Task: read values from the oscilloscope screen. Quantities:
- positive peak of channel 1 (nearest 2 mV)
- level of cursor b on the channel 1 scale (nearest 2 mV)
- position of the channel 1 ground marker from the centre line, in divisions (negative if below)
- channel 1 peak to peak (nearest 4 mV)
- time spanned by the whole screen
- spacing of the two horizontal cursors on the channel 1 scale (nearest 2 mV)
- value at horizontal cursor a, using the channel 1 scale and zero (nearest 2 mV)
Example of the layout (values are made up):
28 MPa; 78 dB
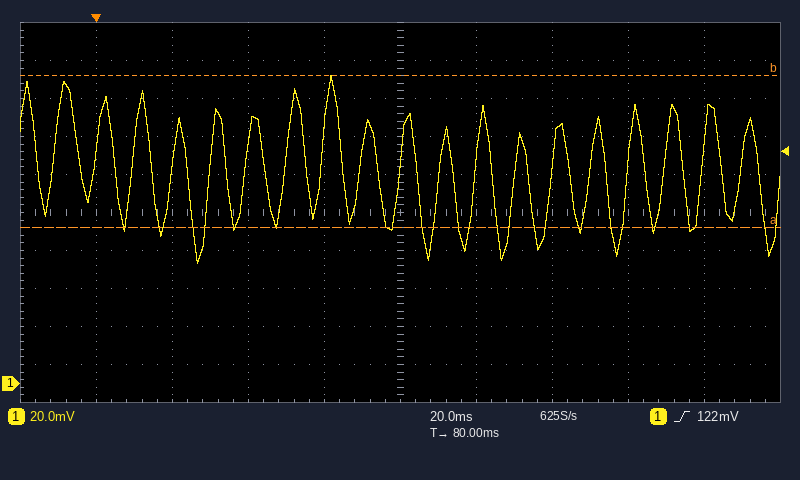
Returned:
162 mV; 162 mV; -4.5 div; 100 mV; 200 ms; 80 mV; 82 mV
